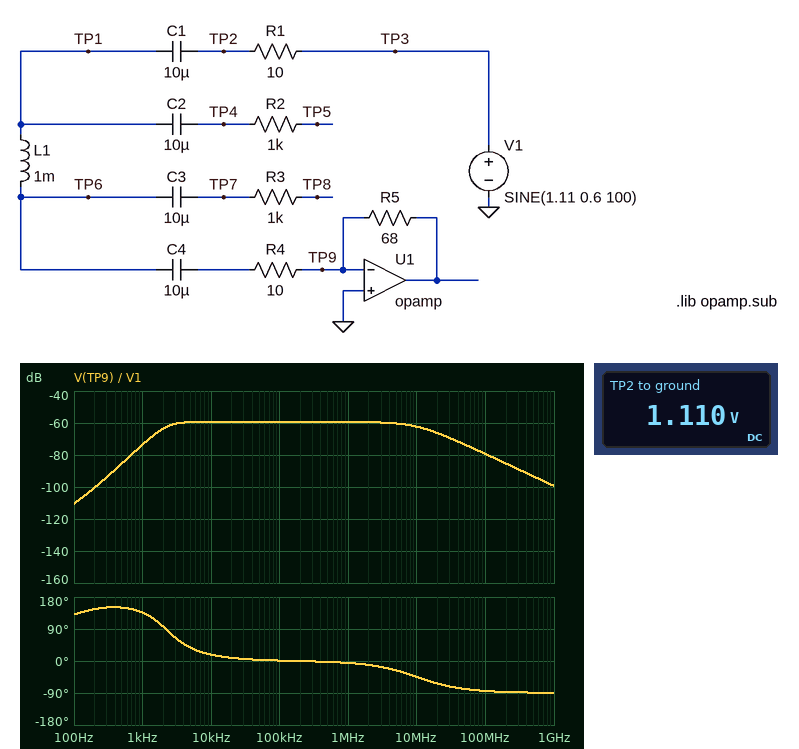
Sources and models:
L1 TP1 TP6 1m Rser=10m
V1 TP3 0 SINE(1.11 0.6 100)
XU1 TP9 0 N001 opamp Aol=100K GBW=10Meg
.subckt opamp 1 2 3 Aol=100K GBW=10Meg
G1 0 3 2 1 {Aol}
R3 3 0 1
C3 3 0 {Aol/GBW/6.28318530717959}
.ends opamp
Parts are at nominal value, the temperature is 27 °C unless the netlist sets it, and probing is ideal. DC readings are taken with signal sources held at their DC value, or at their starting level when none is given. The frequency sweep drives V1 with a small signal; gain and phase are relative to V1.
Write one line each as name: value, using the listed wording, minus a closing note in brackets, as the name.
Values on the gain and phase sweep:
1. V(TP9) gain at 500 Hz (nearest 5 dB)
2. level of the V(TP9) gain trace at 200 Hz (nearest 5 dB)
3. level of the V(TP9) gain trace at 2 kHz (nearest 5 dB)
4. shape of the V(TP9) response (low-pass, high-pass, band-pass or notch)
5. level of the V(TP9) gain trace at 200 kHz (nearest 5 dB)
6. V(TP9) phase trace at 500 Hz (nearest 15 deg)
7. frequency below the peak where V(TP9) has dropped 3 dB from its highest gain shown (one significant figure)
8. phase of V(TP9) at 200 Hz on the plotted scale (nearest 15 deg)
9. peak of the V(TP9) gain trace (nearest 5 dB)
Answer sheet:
V(TP9) gain at 500 Hz: -85 dB
level of the V(TP9) gain trace at 200 Hz: -100 dB
level of the V(TP9) gain trace at 2 kHz: -65 dB
shape of the V(TP9) response: band-pass
level of the V(TP9) gain trace at 200 kHz: -60 dB
V(TP9) phase trace at 500 Hz: 150 deg
frequency below the peak where V(TP9) has dropped 3 dB from its highest gain shown: 2 kHz
phase of V(TP9) at 200 Hz on the plotted scale: 150 deg
peak of the V(TP9) gain trace: -60 dB
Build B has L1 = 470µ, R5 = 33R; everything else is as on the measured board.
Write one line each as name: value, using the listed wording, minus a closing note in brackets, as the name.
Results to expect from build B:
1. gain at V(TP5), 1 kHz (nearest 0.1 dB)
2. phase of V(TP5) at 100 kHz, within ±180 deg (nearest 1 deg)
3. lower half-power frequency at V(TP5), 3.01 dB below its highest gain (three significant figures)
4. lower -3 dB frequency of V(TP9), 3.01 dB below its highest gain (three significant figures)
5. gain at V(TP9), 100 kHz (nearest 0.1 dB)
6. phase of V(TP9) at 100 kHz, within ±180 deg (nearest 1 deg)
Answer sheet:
gain at V(TP5), 1 kHz: -6.6 dB
phase of V(TP5) at 100 kHz, within ±180 deg: 2 deg
lower half-power frequency at V(TP5), 3.01 dB below its highest gain: 5.02 kHz
lower -3 dB frequency of V(TP9), 3.01 dB below its highest gain: 5.32 kHz
gain at V(TP9), 100 kHz: -59.1 dB
phase of V(TP9) at 100 kHz, within ±180 deg: 3 deg
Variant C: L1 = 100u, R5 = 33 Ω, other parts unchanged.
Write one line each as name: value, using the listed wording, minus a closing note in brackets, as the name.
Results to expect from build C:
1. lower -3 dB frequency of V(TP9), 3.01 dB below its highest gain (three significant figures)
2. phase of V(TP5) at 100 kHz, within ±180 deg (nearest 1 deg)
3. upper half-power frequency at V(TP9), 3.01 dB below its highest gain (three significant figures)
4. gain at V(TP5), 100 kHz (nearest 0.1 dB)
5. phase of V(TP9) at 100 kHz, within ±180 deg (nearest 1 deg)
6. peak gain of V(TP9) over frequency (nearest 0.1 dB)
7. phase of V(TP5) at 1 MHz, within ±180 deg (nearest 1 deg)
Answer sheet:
lower -3 dB frequency of V(TP9), 3.01 dB below its highest gain: 29.9 kHz
phase of V(TP5) at 100 kHz, within ±180 deg: 9 deg
upper half-power frequency at V(TP9), 3.01 dB below its highest gain: 10.1 MHz
gain at V(TP5), 100 kHz: -0.3 dB
phase of V(TP9) at 100 kHz, within ±180 deg: 17 deg
peak gain of V(TP9) over frequency: -45.7 dB
phase of V(TP5) at 1 MHz, within ±180 deg: 1 deg
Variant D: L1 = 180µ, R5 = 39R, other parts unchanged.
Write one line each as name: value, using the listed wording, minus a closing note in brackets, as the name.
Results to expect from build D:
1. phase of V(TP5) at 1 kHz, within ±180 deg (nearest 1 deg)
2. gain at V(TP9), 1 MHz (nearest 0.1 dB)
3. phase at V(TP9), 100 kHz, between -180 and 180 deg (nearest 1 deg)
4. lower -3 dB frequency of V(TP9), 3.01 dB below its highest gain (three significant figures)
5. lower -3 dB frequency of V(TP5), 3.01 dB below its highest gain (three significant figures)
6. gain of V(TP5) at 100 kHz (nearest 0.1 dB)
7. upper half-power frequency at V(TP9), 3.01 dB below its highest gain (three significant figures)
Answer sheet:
phase of V(TP5) at 1 kHz, within ±180 deg: 1 deg
gain at V(TP9), 1 MHz: -49.3 dB
phase at V(TP9), 100 kHz, between -180 and 180 deg: 9 deg
lower -3 dB frequency of V(TP9), 3.01 dB below its highest gain: 16.0 kHz
lower -3 dB frequency of V(TP5), 3.01 dB below its highest gain: 12.6 kHz
gain of V(TP5) at 100 kHz: -0.1 dB
upper half-power frequency at V(TP9), 3.01 dB below its highest gain: 10.1 MHz
